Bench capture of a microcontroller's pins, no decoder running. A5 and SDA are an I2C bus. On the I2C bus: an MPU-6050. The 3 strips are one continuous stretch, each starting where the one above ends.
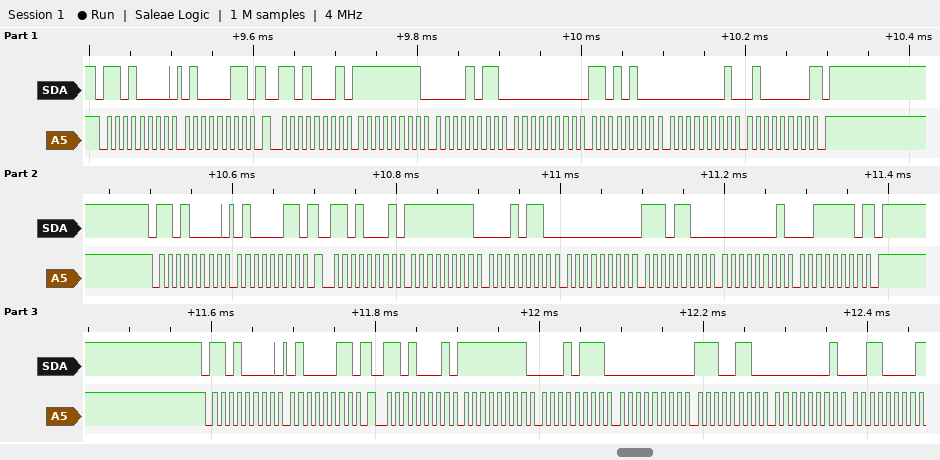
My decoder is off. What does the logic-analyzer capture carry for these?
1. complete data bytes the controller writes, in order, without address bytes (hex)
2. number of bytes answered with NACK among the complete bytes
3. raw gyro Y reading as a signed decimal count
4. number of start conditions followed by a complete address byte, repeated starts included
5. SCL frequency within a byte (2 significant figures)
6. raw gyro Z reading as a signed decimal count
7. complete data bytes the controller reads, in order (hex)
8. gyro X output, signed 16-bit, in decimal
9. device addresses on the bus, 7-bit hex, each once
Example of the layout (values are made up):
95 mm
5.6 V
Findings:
43 43 43
3
212
6
100 kHz
320
FF 0B 00 D4 01 40 FF 16 00 EC 01 3E FF 17 00 E6 01 30
-245
0x68
